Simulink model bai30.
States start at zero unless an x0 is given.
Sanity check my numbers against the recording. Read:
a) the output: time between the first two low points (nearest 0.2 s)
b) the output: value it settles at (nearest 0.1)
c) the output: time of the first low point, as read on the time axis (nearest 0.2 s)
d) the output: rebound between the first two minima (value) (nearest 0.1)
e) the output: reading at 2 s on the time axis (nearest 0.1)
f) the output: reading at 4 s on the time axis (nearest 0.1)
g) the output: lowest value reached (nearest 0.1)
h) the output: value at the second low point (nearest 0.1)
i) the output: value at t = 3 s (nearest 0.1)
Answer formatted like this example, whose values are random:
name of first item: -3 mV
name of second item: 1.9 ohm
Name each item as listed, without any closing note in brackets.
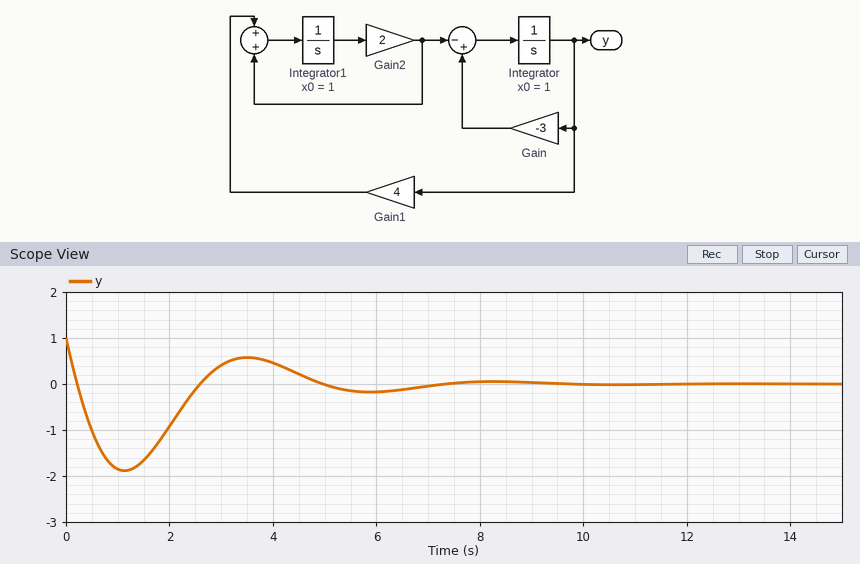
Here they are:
the output: time between the first two low points: 4.8 s
the output: value it settles at: 0.0
the output: time of the first low point, as read on the time axis: 1.2 s
the output: rebound between the first two minima (value): 0.6
the output: reading at 2 s on the time axis: -0.9
the output: reading at 4 s on the time axis: 0.5
the output: lowest value reached: -1.9
the output: value at the second low point: -0.2
the output: value at t = 3 s: 0.4
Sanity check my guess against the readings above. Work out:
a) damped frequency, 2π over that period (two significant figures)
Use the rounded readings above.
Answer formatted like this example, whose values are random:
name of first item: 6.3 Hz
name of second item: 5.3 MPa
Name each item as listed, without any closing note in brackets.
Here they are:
damped frequency, 2π over that period: 1.3 rad/s
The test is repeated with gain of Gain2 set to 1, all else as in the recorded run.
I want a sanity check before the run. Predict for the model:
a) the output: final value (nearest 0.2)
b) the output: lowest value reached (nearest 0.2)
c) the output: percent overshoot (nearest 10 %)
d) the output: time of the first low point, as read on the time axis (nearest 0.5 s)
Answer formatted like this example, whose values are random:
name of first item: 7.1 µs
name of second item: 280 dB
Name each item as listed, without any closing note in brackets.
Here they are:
the output: final value: 0.0
the output: lowest value reached: -0.8
the output: percent overshoot: 80 %
the output: time of the first low point, as read on the time axis: 1.5 s
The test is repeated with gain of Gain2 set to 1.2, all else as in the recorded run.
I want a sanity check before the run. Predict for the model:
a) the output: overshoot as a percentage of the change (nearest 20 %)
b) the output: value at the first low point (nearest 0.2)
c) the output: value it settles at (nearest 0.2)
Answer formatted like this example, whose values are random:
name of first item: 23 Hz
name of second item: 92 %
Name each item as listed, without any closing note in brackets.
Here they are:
the output: overshoot as a percentage of the change: 100 %
the output: value at the first low point: -1.0
the output: value it settles at: 0.0
